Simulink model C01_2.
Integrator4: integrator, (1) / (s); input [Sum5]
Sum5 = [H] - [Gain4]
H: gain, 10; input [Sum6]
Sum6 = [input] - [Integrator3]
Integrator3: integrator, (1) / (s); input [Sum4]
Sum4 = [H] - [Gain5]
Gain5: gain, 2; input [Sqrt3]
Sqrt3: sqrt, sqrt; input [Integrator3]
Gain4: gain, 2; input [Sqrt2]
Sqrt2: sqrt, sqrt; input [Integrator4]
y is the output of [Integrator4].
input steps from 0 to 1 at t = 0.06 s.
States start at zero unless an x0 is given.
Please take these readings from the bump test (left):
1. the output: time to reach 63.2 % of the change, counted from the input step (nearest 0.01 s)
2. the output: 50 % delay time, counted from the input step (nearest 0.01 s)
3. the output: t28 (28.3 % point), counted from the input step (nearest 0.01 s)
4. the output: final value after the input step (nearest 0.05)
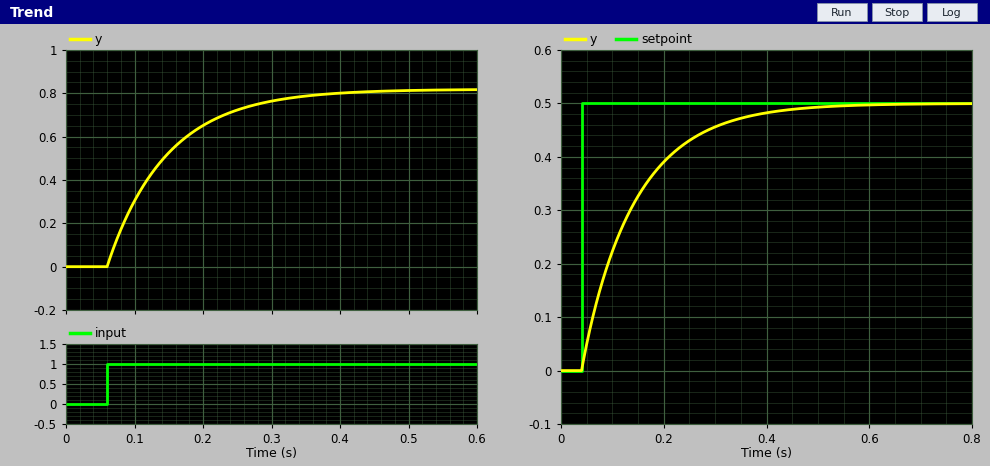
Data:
0.09 s
0.06 s
0.03 s
0.80
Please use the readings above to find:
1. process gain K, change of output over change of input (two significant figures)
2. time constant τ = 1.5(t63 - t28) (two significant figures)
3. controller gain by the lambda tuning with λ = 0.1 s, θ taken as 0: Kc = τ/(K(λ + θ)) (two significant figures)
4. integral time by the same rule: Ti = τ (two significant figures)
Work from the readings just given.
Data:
0.80
0.090 s
1.1
0.090 s
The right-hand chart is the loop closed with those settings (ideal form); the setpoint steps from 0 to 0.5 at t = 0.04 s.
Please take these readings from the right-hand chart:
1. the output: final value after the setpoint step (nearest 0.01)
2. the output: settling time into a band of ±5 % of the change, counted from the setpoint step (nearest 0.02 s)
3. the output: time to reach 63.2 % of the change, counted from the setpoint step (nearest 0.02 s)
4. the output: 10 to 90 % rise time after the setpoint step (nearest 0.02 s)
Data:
0.50
0.32 s
0.10 s
0.24 s
